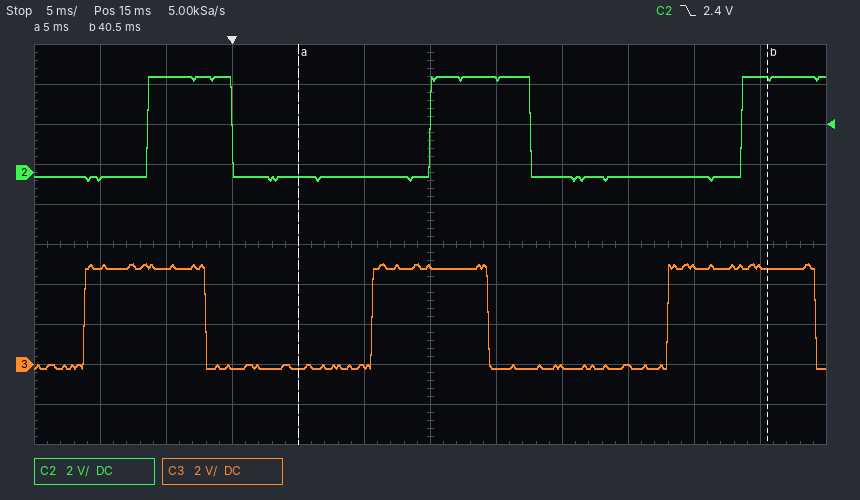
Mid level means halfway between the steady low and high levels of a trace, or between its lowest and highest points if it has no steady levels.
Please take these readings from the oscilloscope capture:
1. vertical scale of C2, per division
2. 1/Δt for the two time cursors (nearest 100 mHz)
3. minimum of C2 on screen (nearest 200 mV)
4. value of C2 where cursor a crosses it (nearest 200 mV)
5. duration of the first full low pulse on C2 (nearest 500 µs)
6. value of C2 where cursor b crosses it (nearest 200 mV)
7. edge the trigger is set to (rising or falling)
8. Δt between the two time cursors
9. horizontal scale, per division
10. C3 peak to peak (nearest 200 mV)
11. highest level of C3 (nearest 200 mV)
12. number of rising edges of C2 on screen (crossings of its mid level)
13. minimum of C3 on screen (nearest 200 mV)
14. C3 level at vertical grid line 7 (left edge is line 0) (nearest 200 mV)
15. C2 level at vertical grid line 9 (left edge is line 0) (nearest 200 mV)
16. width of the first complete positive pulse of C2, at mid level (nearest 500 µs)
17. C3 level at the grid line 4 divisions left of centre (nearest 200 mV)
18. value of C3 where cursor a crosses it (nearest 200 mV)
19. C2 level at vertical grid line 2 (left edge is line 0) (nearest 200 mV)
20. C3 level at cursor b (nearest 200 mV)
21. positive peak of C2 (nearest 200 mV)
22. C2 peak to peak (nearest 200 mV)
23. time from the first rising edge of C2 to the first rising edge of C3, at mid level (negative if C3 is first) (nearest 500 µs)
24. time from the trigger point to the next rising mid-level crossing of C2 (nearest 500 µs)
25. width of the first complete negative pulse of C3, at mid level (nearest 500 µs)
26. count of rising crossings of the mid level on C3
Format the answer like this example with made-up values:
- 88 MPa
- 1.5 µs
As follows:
- 2 V
- 28.2 Hz
- -400 mV
- -200 mV
- 15.0 ms
- 4.8 V
- falling
- 35.5 ms
- 5 ms
- 5.2 V
- 5.0 V
- 3
- -200 mV
- -200 mV
- -200 mV
- 6.5 ms
- 4.8 V
- -200 mV
- 4.8 V
- 4.8 V
- 4.8 V
- 5.2 V
- -5.0 ms
- 15.0 ms
- 12.5 ms
- 3
